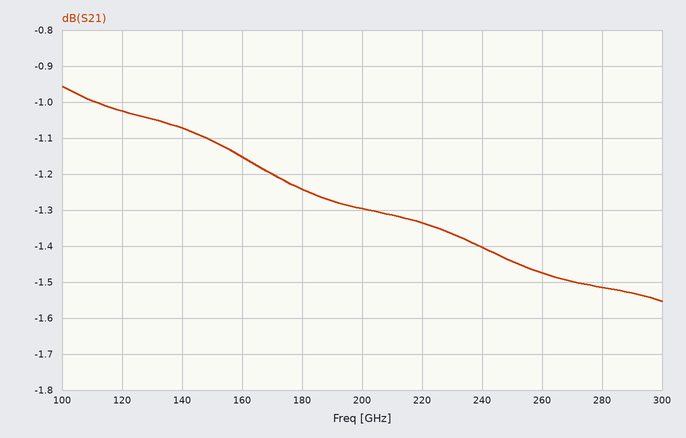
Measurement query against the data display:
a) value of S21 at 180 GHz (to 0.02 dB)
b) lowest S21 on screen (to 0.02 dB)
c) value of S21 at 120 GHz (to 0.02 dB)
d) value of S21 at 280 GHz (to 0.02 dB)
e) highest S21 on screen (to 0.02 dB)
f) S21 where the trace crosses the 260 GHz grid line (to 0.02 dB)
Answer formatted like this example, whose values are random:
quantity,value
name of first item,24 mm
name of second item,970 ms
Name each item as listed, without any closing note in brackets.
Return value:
quantity,value
value of S21 at 180 GHz,-1.24 dB
lowest S21 on screen,-1.56 dB
value of S21 at 120 GHz,-1.02 dB
value of S21 at 280 GHz,-1.52 dB
highest S21 on screen,-0.96 dB
S21 where the trace crosses the 260 GHz grid line,-1.48 dB
